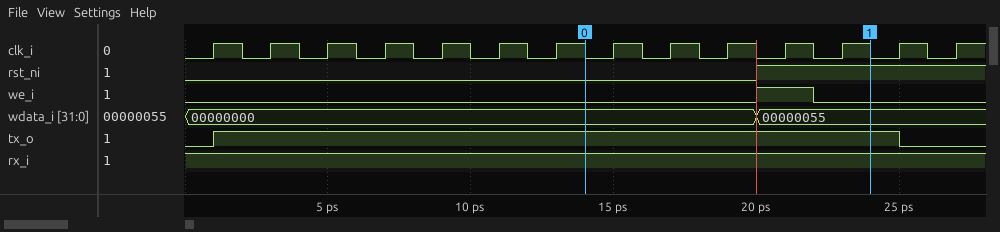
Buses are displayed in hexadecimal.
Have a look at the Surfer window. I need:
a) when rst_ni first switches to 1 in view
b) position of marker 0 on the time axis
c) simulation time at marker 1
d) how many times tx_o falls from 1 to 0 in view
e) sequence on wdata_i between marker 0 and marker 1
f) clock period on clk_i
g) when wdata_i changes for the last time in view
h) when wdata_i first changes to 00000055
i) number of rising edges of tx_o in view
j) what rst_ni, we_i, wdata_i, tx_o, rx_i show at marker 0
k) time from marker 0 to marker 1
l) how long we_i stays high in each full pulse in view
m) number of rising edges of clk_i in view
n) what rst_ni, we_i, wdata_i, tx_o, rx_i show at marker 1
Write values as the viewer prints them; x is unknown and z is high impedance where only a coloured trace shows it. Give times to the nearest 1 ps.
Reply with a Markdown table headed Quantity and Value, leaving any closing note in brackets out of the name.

| Quantity | Value |
|---|---|
| when rst_ni first switches to 1 in view | 20 ps |
| position of marker 0 on the time axis | 14 ps |
| simulation time at marker 1 | 24 ps |
| how many times tx_o falls from 1 to 0 in view | 1 |
| sequence on wdata_i between marker 0 and marker 1 | 00000000, 00000055 |
| clock period on clk_i | 2 ps |
| when wdata_i changes for the last time in view | 20 ps |
| when wdata_i first changes to 00000055 | 20 ps |
| number of rising edges of tx_o in view | 1 |
| what rst_ni, we_i, wdata_i, tx_o, rx_i show at marker 0 | rst_ni=0, we_i=0, wdata_i=00000000, tx_o=1, rx_i=1 |
| time from marker 0 to marker 1 | 10 ps |
| how long we_i stays high in each full pulse in view | 2 ps |
| number of rising edges of clk_i in view | 14 |
| what rst_ni, we_i, wdata_i, tx_o, rx_i show at marker 1 | rst_ni=1, we_i=0, wdata_i=00000055, tx_o=1, rx_i=1 |
